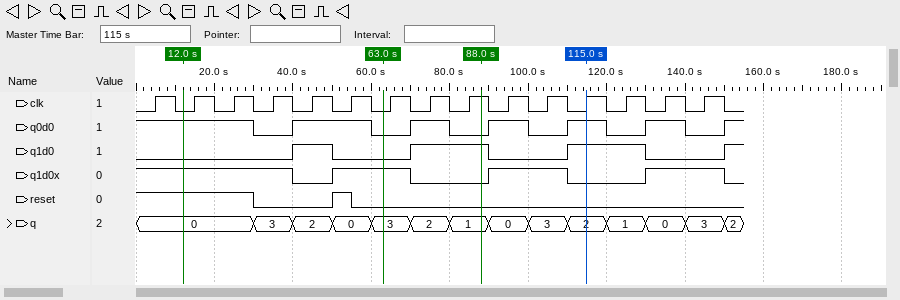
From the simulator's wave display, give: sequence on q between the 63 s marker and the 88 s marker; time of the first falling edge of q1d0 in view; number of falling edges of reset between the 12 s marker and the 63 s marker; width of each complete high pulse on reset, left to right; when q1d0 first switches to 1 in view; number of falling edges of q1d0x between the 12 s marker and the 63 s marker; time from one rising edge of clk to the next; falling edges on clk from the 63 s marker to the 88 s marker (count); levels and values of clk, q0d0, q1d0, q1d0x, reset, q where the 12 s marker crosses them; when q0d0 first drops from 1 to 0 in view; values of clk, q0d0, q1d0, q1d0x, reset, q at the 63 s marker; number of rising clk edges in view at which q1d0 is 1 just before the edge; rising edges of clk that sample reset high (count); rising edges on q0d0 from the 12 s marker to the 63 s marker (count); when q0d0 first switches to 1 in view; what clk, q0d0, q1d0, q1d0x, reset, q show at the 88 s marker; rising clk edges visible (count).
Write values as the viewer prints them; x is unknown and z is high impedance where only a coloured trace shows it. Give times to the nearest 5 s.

3, 2, 1
50 s
2
5 s
40 s
1
10 s
2
clk=0, q0d0=1, q1d0=0, q1d0x=1, reset=1, q=0
30 s
clk=0, q0d0=0, q1d0=0, q1d0x=1, reset=0, q=3
5
4
1
40 s
clk=1, q0d0=0, q1d0=1, q1d0x=0, reset=0, q=1
15
